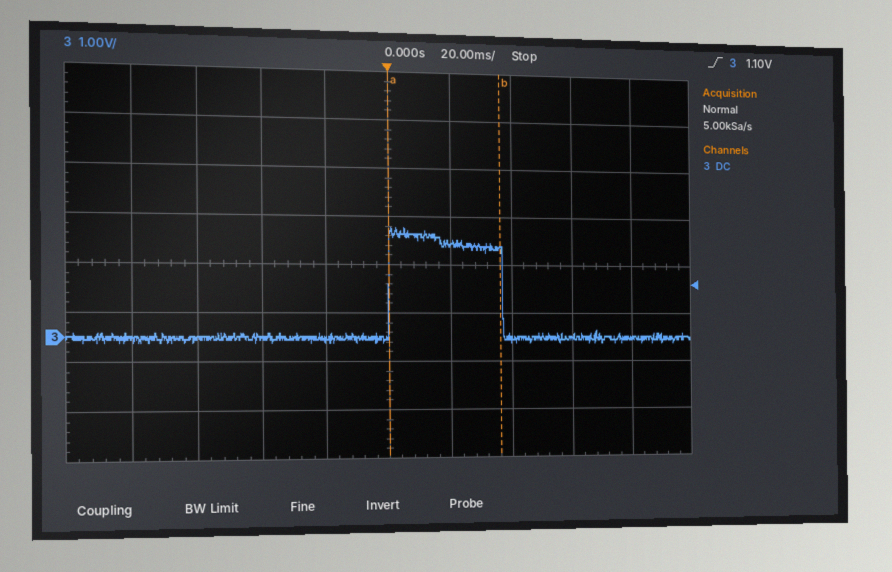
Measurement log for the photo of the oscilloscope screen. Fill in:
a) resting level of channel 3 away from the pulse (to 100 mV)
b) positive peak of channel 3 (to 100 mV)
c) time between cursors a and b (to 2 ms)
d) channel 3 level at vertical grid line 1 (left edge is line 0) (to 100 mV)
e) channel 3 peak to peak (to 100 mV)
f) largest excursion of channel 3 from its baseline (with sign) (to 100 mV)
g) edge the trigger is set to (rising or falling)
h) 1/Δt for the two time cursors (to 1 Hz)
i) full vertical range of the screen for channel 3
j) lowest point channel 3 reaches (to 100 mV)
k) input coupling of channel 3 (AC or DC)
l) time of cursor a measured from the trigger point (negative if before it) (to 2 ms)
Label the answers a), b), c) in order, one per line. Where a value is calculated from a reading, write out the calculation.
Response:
a) 0.0 V
b) 2.3 V
c) 36 ms
d) 0.0 V
e) 2.3 V − (-100 mV) = 2.4 V
f) 2.3 V − (0.0 V) = +2.3 V
g) rising
h) 1 / 36 ms ≈ 28 Hz
i) 8 V
j) -100 mV
k) DC
l) 0 ms
